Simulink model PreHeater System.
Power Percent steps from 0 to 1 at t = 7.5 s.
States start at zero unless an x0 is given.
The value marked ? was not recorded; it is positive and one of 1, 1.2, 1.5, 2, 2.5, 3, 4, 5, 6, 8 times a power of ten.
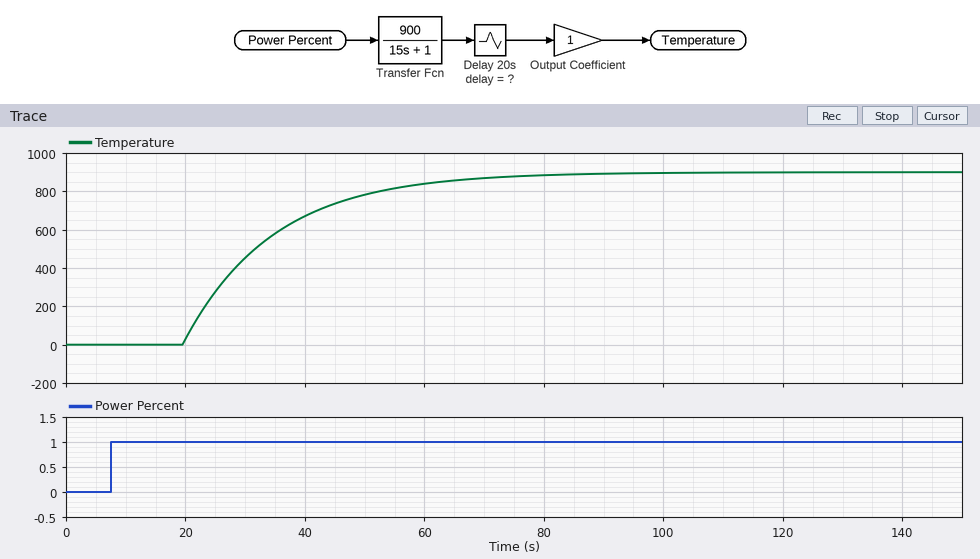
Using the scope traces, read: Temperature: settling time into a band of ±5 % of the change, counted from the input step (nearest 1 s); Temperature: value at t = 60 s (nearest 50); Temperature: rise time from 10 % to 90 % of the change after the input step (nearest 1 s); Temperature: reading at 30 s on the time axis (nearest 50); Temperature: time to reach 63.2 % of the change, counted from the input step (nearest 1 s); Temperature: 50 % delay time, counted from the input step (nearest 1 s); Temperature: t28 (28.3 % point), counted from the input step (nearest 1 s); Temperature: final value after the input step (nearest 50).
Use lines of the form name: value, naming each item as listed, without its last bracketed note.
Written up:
Temperature: settling time into a band of ±5 % of the change, counted from the input step: 57 s
Temperature: value at t = 60 s: 850
Temperature: rise time from 10 % to 90 % of the change after the input step: 33 s
Temperature: reading at 30 s on the time axis: 450
Temperature: time to reach 63.2 % of the change, counted from the input step: 27 s
Temperature: 50 % delay time, counted from the input step: 22 s
Temperature: t28 (28.3 % point), counted from the input step: 17 s
Temperature: final value after the input step: 900
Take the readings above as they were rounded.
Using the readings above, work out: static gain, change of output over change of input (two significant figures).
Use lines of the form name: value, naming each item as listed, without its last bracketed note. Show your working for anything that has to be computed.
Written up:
static gain, change of output over change of input: (900 - 0) / (1 - 0) = 900
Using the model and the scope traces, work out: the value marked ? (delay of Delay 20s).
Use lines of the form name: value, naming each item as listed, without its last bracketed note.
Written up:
the value marked ?: 12
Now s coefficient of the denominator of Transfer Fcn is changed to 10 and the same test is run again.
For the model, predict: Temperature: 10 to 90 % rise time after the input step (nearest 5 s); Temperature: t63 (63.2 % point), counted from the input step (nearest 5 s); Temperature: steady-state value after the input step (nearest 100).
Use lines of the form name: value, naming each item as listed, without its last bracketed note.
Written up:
Temperature: 10 to 90 % rise time after the input step: 20 s
Temperature: t63 (63.2 % point), counted from the input step: 20 s
Temperature: steady-state value after the input step: 900
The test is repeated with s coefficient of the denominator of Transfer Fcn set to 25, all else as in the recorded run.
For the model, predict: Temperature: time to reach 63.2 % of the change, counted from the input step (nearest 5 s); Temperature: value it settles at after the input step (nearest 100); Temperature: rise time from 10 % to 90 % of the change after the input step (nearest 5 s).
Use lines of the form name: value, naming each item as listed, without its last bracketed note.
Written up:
Temperature: time to reach 63.2 % of the change, counted from the input step: 35 s
Temperature: value it settles at after the input step: 900
Temperature: rise time from 10 % to 90 % of the change after the input step: 55 s
